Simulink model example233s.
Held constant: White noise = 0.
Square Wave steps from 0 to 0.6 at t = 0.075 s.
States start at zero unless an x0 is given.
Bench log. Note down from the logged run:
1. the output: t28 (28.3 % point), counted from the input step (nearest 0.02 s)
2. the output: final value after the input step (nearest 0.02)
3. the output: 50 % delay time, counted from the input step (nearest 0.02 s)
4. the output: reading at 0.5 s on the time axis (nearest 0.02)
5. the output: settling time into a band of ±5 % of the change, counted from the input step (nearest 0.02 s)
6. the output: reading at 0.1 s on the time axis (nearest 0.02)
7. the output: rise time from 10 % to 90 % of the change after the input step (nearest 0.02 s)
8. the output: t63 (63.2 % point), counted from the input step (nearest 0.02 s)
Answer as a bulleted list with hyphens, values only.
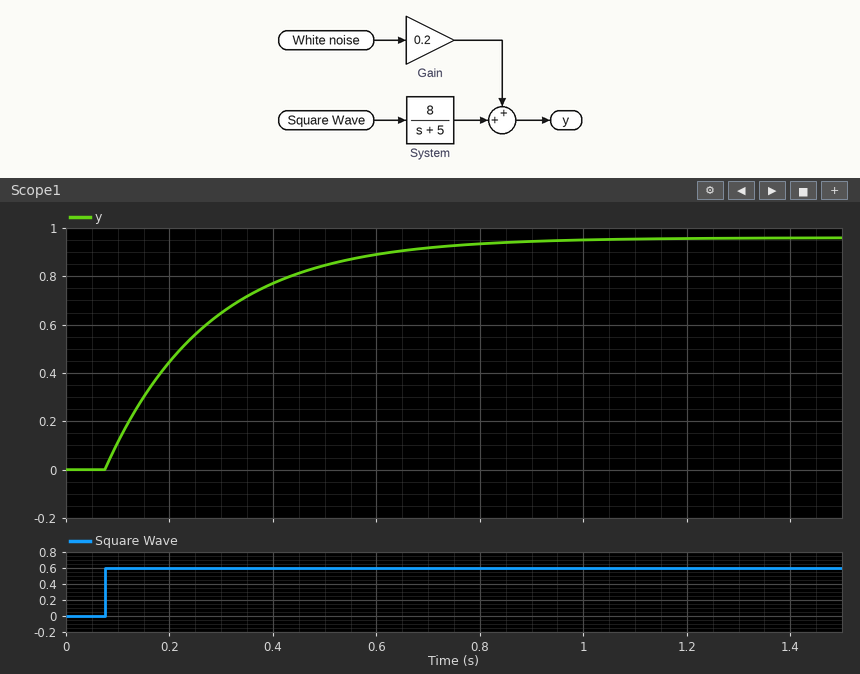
- 0.06 s
- 0.96
- 0.14 s
- 0.84
- 0.60 s
- 0.12
- 0.44 s
- 0.20 s
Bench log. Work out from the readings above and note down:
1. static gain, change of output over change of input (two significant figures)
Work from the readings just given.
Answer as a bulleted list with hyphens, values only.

- 1.6
